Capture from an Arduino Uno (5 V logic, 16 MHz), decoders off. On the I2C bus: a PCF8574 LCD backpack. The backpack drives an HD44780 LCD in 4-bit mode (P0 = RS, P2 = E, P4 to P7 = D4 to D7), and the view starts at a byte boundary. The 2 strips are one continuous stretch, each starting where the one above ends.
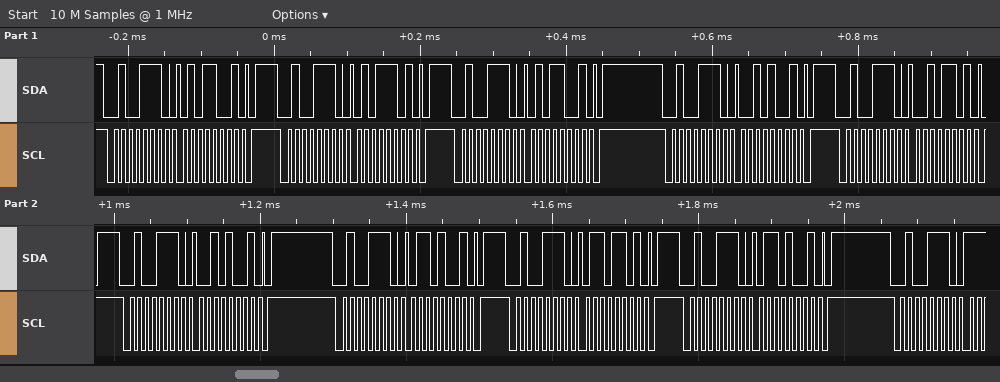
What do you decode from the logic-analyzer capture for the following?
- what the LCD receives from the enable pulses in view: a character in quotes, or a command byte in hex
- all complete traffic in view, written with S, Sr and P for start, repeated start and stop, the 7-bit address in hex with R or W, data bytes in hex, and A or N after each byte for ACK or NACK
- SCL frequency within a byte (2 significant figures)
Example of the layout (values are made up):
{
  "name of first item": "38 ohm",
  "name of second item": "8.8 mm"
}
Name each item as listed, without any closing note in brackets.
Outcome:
{
  "what the LCD receives from the enable pulses in view: a character in quotes, or a command byte in hex": "'R'",
  "all complete traffic in view, written with S, Sr and P for start, repeated start and stop, the 7-bit address in hex with R or W, data bytes in hex, and A or N after each byte for ACK or NACK": "S 27W A 59 A P S 27W A 5D A P S 27W A 59 A P S 27W A 29 A P S 27W A 2D A P S 27W A 29 A P S 27W A 69 A P S 27W A 6D A P S 27W A 69 A P S 27W A",
  "SCL frequency within a byte": "100 kHz"
}
